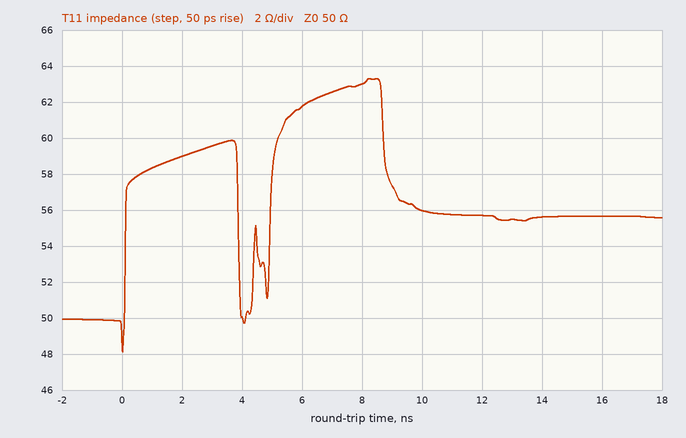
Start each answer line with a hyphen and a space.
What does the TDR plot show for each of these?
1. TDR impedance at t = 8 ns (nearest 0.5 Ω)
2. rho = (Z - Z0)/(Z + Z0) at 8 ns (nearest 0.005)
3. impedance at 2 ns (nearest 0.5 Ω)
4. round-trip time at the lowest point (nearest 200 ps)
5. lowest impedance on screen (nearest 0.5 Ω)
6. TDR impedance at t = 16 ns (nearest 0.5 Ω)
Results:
- 63.0 Ω
- +0.115
- 59.0 Ω
- 0.0 ns
- 48.0 Ω
- 55.5 Ω
